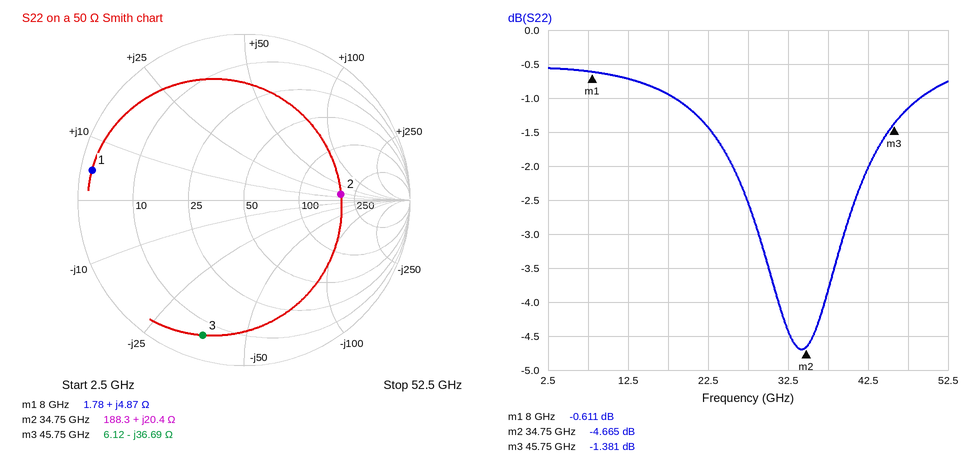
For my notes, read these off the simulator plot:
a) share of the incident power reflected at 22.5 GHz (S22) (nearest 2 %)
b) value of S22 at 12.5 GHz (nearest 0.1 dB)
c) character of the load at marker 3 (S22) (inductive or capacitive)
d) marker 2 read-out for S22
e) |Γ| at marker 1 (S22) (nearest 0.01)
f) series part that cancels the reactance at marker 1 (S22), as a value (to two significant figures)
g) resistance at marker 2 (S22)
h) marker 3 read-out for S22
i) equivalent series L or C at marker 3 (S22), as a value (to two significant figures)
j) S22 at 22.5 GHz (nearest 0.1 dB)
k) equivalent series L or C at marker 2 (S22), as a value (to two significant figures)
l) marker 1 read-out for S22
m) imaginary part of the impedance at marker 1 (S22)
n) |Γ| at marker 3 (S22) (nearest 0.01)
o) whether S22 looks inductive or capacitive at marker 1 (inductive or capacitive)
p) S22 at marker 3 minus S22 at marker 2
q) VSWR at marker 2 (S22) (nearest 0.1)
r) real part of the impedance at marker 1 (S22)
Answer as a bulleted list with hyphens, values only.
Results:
- 72 %
- -0.7 dB
- capacitive
- -4.665 dB
- 0.93
- 4.1 pF
- 188.3 Ω
- -1.381 dB
- 95 fF
- -1.4 dB
- 93 pH
- -0.611 dB
- +4.87 Ω
- 0.85
- inductive
- 3.284 dB
- 3.8
- 1.78 Ω
